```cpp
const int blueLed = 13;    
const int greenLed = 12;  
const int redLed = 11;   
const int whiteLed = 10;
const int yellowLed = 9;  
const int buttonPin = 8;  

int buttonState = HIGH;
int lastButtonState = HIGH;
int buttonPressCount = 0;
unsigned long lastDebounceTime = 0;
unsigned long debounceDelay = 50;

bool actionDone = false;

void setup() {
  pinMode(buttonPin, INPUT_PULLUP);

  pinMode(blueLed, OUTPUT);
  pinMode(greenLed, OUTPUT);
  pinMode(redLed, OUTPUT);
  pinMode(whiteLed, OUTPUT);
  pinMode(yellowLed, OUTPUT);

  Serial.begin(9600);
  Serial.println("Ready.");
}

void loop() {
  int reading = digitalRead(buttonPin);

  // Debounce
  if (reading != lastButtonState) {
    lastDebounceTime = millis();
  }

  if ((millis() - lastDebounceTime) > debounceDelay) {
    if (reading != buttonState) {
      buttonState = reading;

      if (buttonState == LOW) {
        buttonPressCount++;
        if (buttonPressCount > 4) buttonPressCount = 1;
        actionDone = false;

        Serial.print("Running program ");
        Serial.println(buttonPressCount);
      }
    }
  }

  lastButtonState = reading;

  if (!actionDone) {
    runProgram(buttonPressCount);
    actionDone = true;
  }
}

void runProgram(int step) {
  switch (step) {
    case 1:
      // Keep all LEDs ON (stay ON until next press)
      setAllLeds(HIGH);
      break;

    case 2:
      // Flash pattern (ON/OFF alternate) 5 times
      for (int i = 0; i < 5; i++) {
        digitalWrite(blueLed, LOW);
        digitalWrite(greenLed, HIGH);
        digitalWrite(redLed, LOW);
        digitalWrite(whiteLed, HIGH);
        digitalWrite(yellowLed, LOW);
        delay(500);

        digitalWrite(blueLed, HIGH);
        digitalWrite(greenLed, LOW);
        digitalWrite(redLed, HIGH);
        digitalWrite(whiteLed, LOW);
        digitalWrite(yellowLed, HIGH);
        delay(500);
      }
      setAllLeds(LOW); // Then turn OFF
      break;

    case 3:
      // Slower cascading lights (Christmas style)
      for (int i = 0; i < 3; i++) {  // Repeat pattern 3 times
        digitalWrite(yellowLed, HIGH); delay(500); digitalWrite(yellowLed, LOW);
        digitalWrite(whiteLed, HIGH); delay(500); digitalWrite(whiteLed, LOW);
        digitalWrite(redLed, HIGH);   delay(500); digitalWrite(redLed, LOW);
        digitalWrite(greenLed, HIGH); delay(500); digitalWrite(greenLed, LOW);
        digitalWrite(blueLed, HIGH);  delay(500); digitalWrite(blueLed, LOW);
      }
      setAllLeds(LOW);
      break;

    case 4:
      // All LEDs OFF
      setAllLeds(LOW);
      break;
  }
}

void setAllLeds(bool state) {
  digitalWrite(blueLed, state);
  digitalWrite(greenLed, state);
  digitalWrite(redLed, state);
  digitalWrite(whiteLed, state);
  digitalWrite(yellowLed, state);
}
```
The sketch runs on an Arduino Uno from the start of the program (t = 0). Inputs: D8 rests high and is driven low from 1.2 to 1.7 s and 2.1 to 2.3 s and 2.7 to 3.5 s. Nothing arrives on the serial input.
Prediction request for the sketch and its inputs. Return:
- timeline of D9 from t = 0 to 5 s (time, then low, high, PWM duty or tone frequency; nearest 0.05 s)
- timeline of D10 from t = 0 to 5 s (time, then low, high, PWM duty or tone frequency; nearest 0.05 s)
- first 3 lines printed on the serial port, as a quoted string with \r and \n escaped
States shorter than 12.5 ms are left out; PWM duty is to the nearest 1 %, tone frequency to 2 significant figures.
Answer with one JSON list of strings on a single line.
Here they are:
["0 s low; 1.25 s high; 2.15 s low; 2.65 s high; 3.15 s low; 3.65 s high; 4.15 s low; 4.65 s high", "0 s low; 1.25 s high; 2.65 s low; 3.15 s high; 3.65 s low; 4.15 s high; 4.65 s low", "\"Ready.\\r\\nRunning program 1\\r\\nRunning program 2\\r\\n\""]
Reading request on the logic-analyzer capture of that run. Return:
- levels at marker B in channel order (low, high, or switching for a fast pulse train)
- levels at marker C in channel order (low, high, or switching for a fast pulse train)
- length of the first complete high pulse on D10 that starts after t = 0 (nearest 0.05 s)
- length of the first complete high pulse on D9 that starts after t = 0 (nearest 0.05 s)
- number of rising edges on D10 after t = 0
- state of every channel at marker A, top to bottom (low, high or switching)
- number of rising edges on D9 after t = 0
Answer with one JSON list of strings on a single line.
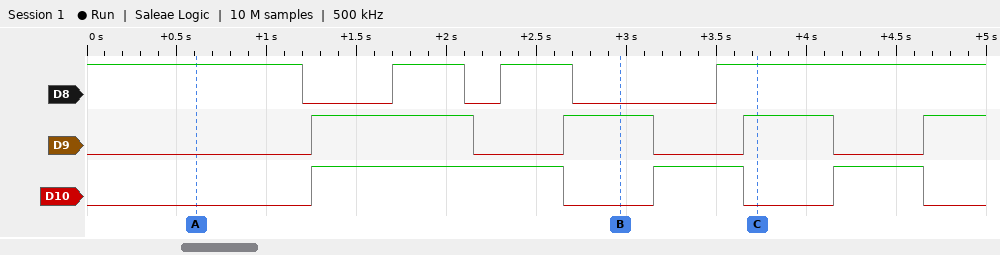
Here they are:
["D8 low, D9 high, D10 low", "D8 high, D9 high, D10 low", "1.40 s", "0.90 s", "3", "D8 high, D9 low, D10 low", "4"]
